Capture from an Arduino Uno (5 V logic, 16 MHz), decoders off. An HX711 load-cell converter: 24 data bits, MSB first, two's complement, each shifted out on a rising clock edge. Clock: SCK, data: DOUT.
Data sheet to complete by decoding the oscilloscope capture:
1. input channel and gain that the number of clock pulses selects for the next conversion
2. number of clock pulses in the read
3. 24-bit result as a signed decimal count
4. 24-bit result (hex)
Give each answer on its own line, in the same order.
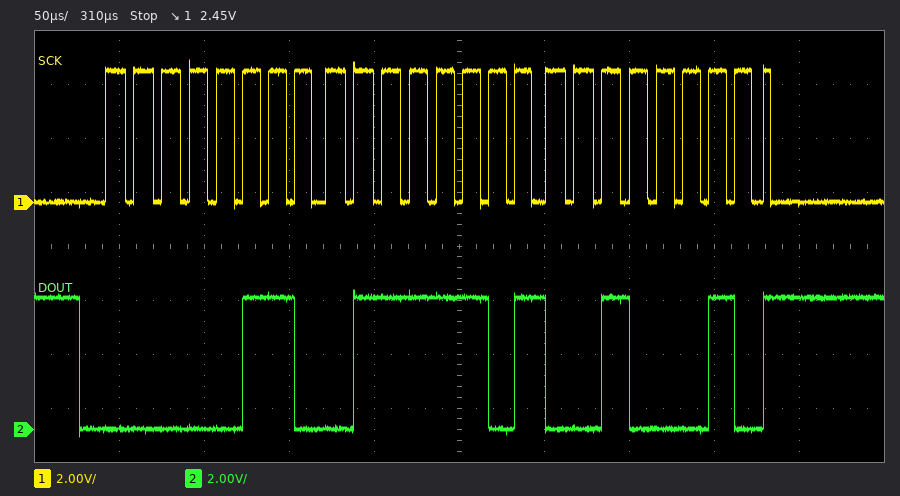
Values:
channel A, gain 128
25
425250
0x067D22
